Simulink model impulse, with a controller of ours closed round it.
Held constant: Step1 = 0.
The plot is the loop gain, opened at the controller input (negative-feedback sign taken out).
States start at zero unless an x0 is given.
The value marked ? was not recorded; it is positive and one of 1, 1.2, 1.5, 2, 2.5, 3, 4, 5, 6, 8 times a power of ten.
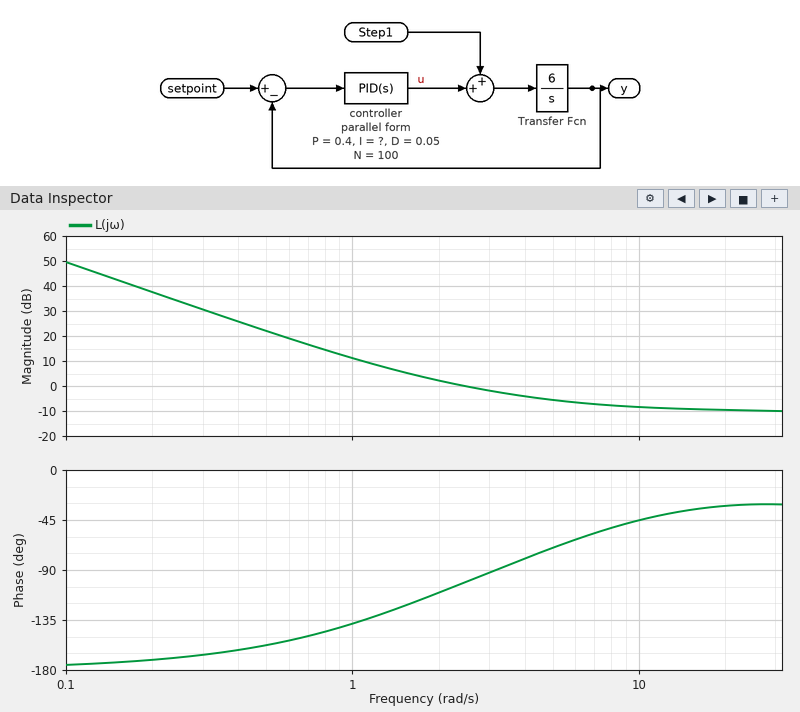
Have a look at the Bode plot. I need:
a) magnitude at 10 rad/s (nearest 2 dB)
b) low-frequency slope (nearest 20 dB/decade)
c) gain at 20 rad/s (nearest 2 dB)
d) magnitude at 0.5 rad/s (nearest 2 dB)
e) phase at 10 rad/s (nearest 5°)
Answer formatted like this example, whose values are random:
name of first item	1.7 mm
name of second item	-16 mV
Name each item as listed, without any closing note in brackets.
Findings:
magnitude at 10 rad/s	-8 dB
low-frequency slope	-40 dB/decade
gain at 20 rad/s	-10 dB
magnitude at 0.5 rad/s	22 dB
phase at 10 rad/s	-45°
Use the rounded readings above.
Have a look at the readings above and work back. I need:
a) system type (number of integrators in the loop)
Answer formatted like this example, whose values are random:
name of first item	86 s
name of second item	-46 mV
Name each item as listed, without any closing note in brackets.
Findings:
system type	2
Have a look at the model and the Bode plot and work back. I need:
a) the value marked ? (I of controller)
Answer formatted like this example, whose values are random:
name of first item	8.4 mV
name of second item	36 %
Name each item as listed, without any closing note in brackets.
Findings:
the value marked ?	0.5
